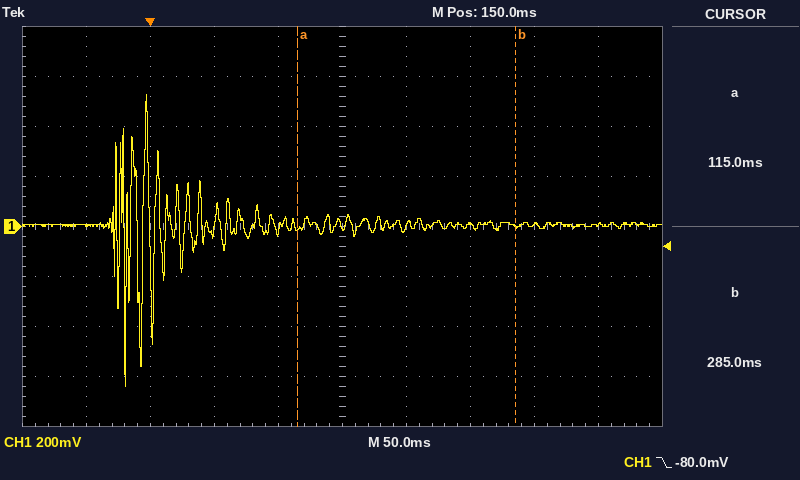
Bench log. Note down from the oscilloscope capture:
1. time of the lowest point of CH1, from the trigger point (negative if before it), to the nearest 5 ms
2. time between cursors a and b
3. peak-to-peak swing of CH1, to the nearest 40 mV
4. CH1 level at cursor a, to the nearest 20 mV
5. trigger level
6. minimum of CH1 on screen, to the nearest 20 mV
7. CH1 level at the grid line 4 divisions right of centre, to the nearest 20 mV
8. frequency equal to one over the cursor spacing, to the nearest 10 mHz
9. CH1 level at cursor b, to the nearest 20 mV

-20 ms
170 ms
1.16 V
0 mV
-80.0 mV
-640 mV
0 mV
5.88 Hz
0 mV
